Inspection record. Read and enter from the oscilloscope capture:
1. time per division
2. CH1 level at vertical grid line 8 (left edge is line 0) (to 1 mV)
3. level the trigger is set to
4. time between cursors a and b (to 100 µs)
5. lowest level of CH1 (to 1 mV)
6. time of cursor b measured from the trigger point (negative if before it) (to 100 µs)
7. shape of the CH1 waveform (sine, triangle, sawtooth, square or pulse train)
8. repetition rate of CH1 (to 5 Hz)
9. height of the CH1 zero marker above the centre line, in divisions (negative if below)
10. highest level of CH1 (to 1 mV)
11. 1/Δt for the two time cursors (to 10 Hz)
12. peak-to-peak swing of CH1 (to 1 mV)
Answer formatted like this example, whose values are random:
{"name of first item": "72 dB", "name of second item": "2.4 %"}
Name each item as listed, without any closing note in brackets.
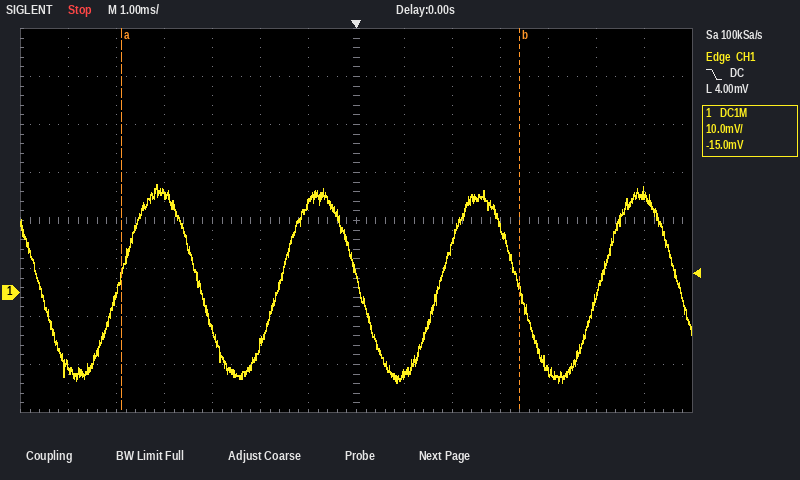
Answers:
{"time per division": "1 ms", "CH1 level at vertical grid line 8 (left edge is line 0)": "-17 mV", "level the trigger is set to": "4.00 mV", "time between cursors a and b": "8.3 ms", "lowest level of CH1": "-19 mV", "time of cursor b measured from the trigger point (negative if before it)": "+3.4 ms", "shape of the CH1 waveform": "sine", "repetition rate of CH1": "300 Hz", "height of the CH1 zero marker above the centre line, in divisions": "-1.5 div", "highest level of CH1": "22 mV", "1/Δt for the two time cursors": "120 Hz", "peak-to-peak swing of CH1": "41 mV"}
